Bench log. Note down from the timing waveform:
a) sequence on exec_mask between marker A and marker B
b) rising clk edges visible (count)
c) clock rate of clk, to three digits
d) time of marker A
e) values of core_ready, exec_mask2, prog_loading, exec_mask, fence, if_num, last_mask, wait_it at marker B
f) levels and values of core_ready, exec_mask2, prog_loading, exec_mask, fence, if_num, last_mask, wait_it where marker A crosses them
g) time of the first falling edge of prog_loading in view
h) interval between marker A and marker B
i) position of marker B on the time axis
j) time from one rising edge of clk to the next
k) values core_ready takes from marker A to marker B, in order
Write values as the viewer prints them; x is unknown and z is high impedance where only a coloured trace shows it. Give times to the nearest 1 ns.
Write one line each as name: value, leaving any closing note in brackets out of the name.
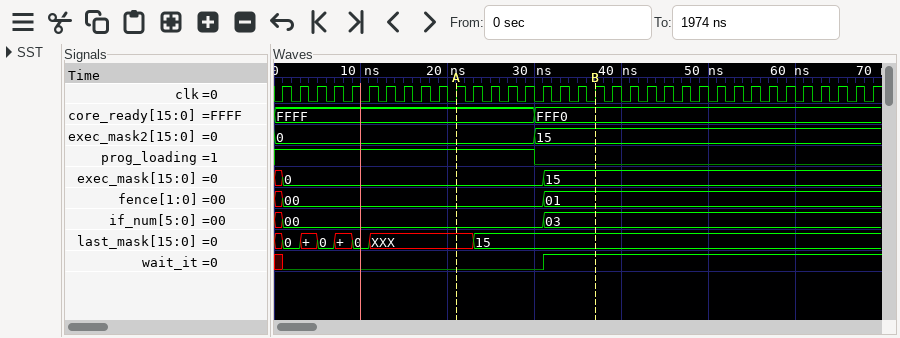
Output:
sequence on exec_mask between marker A and marker B: 0, 15
rising clk edges visible: 35
clock rate of clk, to three digits: 500 MHz
time of marker A: 21 ns
values of core_ready, exec_mask2, prog_loading, exec_mask, fence, if_num, last_mask, wait_it at marker B: core_ready=FFF0, exec_mask2=15, prog_loading=0, exec_mask=15, fence=01, if_num=03, last_mask=15, wait_it=1
levels and values of core_ready, exec_mask2, prog_loading, exec_mask, fence, if_num, last_mask, wait_it where marker A crosses them: core_ready=FFFF, exec_mask2=0, prog_loading=1, exec_mask=0, fence=00, if_num=00, last_mask=XXX, wait_it=0
time of the first falling edge of prog_loading in view: 30 ns
interval between marker A and marker B: 16 ns
position of marker B on the time axis: 37 ns
time from one rising edge of clk to the next: 2 ns
values core_ready takes from marker A to marker B, in order: FFFF, FFF0
